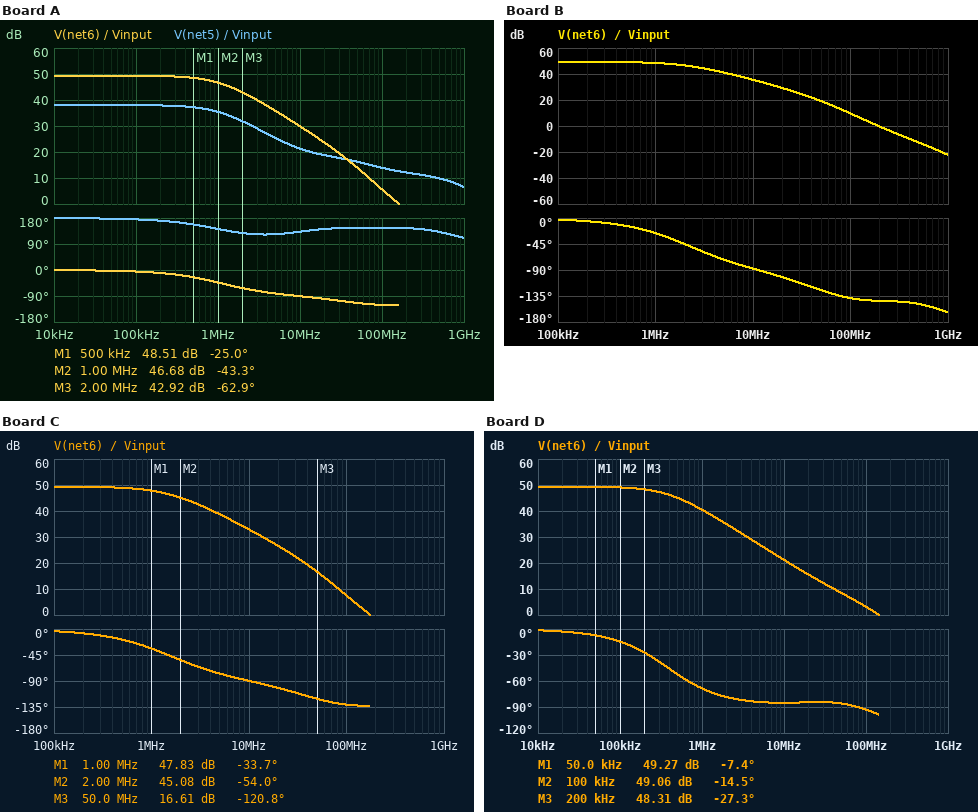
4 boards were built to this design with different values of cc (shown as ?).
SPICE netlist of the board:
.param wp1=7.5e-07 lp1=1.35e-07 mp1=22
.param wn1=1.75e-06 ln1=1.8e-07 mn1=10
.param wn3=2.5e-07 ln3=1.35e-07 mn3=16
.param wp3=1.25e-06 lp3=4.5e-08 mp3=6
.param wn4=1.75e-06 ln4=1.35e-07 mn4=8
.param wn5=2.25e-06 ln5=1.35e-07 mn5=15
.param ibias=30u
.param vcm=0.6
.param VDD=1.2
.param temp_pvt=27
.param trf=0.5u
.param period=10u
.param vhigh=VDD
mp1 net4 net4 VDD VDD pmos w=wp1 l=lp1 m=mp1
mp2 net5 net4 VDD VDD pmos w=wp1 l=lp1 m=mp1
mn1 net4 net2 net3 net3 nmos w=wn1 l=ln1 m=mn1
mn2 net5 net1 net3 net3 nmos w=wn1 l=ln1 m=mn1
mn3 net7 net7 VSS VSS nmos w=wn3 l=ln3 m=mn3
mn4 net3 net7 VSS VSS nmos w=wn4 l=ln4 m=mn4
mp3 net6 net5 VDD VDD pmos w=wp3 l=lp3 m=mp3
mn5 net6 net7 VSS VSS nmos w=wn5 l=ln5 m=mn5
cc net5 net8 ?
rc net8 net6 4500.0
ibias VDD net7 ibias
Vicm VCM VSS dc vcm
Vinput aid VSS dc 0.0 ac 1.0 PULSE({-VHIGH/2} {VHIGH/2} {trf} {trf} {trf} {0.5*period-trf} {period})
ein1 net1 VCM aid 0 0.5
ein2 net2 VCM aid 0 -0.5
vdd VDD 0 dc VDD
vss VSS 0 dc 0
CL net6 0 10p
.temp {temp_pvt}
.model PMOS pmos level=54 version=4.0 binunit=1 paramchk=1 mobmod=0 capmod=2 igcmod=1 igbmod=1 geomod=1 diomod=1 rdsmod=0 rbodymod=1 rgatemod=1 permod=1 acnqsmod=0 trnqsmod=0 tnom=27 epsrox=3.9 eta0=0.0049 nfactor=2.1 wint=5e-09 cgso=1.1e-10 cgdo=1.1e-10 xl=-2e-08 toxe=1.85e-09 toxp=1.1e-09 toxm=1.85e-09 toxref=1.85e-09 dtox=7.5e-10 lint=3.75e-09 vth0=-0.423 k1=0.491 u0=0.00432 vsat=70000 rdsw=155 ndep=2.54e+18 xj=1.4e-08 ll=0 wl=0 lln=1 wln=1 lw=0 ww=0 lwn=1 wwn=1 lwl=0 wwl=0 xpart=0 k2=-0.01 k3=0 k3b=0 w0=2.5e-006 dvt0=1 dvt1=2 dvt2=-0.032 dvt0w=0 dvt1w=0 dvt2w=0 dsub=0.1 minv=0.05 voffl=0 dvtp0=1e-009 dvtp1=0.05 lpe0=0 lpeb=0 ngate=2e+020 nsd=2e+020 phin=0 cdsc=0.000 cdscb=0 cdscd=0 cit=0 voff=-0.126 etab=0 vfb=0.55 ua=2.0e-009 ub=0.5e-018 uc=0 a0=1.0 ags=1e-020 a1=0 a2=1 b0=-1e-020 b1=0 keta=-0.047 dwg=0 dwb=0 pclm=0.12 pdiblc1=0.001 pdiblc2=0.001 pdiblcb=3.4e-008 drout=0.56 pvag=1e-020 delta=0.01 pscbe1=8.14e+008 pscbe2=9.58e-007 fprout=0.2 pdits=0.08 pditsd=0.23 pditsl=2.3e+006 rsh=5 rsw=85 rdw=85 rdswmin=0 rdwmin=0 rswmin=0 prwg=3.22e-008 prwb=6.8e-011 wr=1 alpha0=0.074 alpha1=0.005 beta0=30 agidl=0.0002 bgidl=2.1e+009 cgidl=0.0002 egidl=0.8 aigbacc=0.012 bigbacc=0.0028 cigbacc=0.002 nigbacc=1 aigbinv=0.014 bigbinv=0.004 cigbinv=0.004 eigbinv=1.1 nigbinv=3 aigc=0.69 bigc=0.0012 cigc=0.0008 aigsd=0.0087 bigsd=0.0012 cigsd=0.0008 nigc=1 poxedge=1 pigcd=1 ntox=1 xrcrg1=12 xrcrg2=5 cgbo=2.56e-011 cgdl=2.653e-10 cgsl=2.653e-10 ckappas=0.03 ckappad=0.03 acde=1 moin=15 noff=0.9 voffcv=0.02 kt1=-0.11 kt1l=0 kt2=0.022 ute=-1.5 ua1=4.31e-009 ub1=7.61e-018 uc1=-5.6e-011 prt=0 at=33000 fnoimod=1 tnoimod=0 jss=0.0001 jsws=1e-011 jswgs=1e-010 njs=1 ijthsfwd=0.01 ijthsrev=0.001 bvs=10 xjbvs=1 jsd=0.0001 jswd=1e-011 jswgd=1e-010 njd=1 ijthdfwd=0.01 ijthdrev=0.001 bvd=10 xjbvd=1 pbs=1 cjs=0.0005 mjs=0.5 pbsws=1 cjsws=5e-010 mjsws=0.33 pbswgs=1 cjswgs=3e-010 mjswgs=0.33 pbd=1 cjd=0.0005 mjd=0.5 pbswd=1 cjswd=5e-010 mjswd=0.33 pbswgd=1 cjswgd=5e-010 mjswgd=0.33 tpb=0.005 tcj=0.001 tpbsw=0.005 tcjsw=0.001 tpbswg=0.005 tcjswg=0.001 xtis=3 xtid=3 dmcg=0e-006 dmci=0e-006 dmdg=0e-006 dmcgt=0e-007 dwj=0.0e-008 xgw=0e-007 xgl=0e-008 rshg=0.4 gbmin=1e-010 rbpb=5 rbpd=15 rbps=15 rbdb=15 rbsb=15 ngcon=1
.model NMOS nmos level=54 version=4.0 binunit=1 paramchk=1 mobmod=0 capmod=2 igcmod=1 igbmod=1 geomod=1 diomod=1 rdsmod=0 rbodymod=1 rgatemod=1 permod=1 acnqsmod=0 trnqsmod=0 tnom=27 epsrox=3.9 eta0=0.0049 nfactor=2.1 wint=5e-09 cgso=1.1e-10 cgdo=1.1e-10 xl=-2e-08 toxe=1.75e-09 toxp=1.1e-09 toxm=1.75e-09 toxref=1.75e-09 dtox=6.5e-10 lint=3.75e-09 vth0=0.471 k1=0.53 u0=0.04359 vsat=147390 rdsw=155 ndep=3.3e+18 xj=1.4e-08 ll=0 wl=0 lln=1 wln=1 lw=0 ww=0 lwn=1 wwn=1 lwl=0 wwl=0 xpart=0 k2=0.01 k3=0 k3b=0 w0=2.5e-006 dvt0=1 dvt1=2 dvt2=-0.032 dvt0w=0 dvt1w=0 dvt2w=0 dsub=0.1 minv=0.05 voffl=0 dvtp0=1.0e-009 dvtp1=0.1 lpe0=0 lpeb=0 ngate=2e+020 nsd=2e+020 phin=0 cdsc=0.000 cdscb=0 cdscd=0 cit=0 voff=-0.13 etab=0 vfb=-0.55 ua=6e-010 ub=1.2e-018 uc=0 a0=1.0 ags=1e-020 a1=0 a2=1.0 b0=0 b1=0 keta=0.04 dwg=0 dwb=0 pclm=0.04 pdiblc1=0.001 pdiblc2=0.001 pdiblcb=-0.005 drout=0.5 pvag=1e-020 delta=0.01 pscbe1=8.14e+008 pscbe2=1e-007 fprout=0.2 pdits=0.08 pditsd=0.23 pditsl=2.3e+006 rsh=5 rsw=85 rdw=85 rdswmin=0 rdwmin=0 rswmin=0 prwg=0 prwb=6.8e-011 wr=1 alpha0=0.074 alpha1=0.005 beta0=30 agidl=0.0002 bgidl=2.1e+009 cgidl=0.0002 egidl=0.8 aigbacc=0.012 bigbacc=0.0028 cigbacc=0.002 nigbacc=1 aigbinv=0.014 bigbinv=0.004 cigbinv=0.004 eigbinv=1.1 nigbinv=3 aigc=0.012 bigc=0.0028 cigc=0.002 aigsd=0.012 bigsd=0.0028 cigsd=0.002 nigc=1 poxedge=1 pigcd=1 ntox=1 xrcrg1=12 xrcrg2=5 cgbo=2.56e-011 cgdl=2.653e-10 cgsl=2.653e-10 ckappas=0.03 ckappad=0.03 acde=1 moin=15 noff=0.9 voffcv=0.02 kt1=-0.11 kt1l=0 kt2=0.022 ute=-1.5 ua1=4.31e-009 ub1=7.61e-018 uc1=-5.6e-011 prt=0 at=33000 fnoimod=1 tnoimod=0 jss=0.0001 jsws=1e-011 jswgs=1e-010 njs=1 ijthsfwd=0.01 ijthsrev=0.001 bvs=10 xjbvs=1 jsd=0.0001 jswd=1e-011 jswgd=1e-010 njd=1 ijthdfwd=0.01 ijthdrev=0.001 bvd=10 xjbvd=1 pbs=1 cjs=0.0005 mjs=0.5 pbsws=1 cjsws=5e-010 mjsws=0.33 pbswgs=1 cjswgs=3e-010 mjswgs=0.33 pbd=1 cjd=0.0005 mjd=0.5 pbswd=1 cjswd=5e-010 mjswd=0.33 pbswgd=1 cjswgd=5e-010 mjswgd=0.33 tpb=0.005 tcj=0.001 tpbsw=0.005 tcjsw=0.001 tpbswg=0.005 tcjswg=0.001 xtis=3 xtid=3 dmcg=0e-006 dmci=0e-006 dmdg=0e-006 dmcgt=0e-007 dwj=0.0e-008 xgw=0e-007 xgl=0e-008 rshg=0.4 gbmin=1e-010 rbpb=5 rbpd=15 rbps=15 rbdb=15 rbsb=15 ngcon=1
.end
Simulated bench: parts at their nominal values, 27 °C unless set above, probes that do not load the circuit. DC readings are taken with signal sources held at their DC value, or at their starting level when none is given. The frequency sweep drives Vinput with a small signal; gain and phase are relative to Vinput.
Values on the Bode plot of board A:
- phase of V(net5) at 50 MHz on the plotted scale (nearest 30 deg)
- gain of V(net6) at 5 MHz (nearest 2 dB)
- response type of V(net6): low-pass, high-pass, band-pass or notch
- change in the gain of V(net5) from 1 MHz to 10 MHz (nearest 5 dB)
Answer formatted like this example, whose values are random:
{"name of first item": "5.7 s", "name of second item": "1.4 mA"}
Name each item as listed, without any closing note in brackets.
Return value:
{"phase of V(net5) at 50 MHz on the plotted scale": "150 deg", "gain of V(net6) at 5 MHz": "36 dB", "response type of V(net6): low-pass, high-pass, band-pass or notch": "low-pass", "change in the gain of V(net5) from 1 MHz to 10 MHz": "-15 dB"}
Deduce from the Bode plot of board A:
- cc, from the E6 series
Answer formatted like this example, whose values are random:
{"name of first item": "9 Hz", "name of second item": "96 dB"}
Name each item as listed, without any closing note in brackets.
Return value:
{"cc, from the E6 series": "330 fF"}
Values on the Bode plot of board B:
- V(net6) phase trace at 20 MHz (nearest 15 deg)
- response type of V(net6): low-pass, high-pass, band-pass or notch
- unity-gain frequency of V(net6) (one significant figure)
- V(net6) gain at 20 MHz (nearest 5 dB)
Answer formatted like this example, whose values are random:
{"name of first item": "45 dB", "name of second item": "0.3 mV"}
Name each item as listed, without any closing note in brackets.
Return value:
{"V(net6) phase trace at 20 MHz": "-105 deg", "response type of V(net6): low-pass, high-pass, band-pass or notch": "low-pass", "unity-gain frequency of V(net6)": "200 MHz", "V(net6) gain at 20 MHz": "30 dB"}
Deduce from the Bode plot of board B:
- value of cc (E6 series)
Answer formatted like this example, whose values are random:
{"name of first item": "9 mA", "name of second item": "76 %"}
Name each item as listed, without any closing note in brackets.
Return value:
{"value of cc": "150 fF"}
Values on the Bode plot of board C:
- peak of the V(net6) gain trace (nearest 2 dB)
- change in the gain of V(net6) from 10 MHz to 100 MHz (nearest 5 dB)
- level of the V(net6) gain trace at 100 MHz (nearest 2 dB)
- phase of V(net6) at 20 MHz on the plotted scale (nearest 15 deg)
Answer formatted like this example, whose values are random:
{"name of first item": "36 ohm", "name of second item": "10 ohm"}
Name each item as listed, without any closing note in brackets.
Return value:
{"peak of the V(net6) gain trace": "50 dB", "change in the gain of V(net6) from 10 MHz to 100 MHz": "-25 dB", "level of the V(net6) gain trace at 100 MHz": "8 dB", "phase of V(net6) at 20 MHz on the plotted scale": "-105 deg"}
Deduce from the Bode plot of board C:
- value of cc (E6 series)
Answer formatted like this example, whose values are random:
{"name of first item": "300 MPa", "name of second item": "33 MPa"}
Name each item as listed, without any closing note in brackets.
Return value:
{"value of cc": "220 fF"}
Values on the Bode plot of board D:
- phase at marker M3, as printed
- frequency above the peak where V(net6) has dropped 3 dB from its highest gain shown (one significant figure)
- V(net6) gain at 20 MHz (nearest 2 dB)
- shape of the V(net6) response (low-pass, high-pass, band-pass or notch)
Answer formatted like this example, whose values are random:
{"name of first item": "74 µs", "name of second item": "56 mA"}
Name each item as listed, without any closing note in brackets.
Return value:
{"phase at marker M3, as printed": "-27.3 deg", "frequency above the peak where V(net6) has dropped 3 dB from its highest gain shown": "400 kHz", "V(net6) gain at 20 MHz": "16 dB", "shape of the V(net6) response": "low-pass"}
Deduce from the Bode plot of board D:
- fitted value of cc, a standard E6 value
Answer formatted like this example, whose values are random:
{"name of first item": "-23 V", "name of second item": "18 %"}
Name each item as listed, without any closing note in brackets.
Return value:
{"fitted value of cc, a standard E6 value": "1 pF"}
